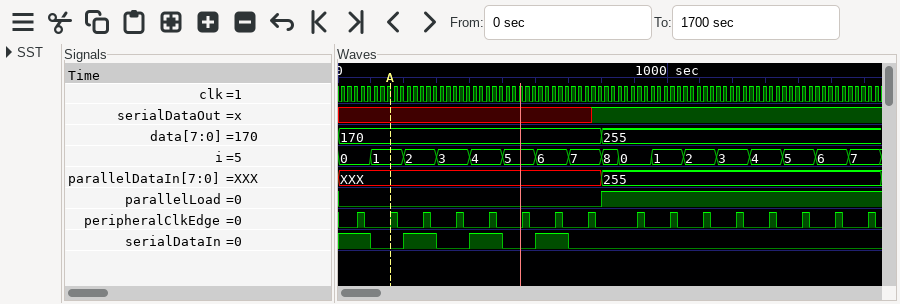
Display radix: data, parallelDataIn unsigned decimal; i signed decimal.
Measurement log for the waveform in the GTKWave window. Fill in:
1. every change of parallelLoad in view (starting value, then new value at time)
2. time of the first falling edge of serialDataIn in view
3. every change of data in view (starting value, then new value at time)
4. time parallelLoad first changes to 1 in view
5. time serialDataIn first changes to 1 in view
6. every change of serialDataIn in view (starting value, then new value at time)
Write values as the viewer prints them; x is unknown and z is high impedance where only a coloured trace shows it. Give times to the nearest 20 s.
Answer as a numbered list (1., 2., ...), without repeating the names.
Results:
1. 0, 1 at 800 s
2. 100 s
3. 170, 255 at 800 s
4. 800 s
5. 200 s
6. 1, 0 at 100 s, 1 at 200 s, 0 at 300 s, 1 at 400 s, 0 at 500 s, 1 at 600 s, 0 at 700 s
